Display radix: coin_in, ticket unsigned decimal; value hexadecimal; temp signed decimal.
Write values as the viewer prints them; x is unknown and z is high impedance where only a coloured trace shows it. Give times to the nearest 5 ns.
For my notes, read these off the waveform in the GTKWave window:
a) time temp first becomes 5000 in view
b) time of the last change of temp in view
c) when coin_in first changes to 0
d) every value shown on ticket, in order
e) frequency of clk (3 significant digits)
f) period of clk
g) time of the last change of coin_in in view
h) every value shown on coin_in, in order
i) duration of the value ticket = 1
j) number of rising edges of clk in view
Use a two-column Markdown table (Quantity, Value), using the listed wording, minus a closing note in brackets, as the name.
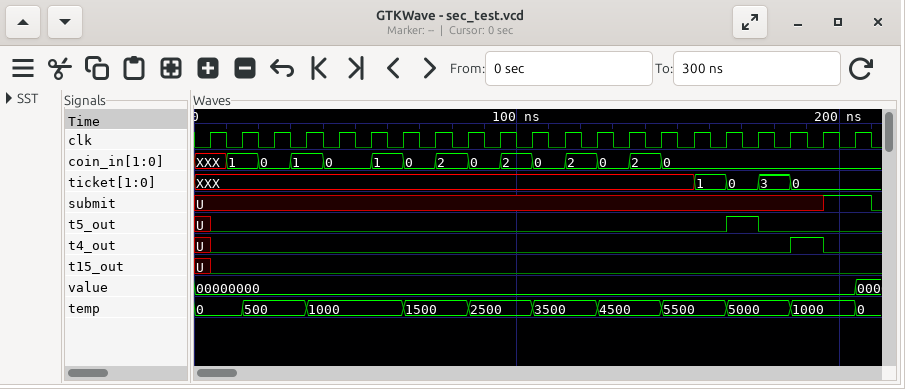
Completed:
| Quantity | Value |
|---|---|
| time temp first becomes 5000 in view | 165 ns |
| time of the last change of temp in view | 205 ns |
| when coin_in first changes to 0 | 20 ns |
| every value shown on ticket, in order | XXX, 1, 0, 3, 0 |
| frequency of clk | 100 MHz |
| period of clk | 10 ns |
| time of the last change of coin_in in view | 145 ns |
| every value shown on coin_in, in order | XXX, 1, 0, 1, 0, 1, 0, 2, 0, 2, 0, 2, 0, 2, 0 |
| duration of the value ticket = 1 | 10 ns |
| number of rising edges of clk in view | 21 |
